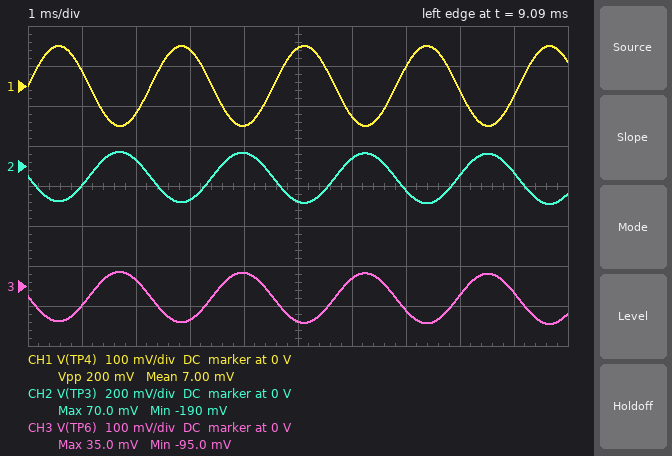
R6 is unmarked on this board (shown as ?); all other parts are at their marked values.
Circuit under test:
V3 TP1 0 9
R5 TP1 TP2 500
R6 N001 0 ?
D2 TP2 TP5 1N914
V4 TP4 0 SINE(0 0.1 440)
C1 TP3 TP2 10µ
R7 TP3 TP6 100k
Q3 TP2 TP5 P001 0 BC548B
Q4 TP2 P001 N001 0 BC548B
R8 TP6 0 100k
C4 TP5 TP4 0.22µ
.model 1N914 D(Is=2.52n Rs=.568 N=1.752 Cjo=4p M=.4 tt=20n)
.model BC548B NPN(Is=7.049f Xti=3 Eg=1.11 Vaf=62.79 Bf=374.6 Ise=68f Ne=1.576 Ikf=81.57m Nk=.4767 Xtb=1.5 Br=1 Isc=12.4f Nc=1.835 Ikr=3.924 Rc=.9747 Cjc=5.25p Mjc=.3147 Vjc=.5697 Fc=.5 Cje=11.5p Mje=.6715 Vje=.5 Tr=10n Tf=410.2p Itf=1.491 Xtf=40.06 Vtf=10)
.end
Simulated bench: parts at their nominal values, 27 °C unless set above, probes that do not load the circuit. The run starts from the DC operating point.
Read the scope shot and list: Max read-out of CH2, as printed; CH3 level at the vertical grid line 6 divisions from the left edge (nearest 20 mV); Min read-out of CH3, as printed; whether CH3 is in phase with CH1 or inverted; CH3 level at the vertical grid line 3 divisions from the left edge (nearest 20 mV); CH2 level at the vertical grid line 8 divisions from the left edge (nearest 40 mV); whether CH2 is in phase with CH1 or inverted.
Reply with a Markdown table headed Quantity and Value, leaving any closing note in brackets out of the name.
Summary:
| Quantity | Value |
|---|---|
| Max read-out of CH2, as printed | 70.0 mV |
| CH3 level at the vertical grid line 6 divisions from the left edge | 20 mV |
| Min read-out of CH3, as printed | -95.0 mV |
| whether CH3 is in phase with CH1 or inverted | inverted |
| CH3 level at the vertical grid line 3 divisions from the left edge | -80 mV |
| CH2 level at the vertical grid line 8 divisions from the left edge | -40 mV |
| whether CH2 is in phase with CH1 or inverted | inverted |
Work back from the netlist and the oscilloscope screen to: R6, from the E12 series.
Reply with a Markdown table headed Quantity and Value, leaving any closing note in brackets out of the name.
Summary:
| Quantity | Value |
|---|---|
| R6, from the E12 series | 390 Ω |
